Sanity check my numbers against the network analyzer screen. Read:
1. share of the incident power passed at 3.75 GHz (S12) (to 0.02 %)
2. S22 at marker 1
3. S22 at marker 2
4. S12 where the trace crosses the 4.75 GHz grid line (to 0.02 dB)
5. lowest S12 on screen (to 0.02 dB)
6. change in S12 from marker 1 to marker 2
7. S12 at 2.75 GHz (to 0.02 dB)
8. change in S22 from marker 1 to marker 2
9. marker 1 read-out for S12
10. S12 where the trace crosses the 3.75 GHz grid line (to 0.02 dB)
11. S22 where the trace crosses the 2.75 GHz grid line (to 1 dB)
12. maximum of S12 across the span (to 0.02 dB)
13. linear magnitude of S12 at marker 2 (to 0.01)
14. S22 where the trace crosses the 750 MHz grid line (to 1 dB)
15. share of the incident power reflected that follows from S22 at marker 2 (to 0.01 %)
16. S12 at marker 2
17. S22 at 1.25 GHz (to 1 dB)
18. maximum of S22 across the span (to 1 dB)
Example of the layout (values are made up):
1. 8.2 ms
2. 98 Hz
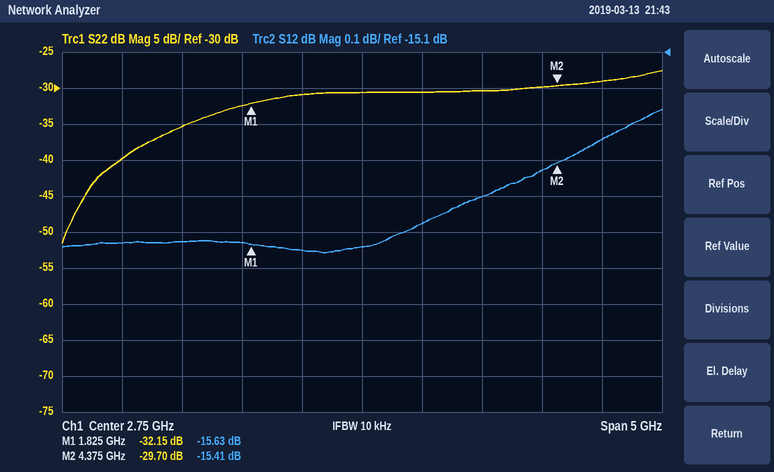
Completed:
1. 2.82 %
2. -32.15 dB
3. -29.70 dB
4. -15.34 dB
5. -15.66 dB
6. 0.22 dB
7. -15.64 dB
8. 2.45 dB
9. -15.63 dB
10. -15.50 dB
11. -31 dB
12. -15.26 dB
13. 0.17
14. -40 dB
15. 0.11 %
16. -15.41 dB
17. -35 dB
18. -28 dB
